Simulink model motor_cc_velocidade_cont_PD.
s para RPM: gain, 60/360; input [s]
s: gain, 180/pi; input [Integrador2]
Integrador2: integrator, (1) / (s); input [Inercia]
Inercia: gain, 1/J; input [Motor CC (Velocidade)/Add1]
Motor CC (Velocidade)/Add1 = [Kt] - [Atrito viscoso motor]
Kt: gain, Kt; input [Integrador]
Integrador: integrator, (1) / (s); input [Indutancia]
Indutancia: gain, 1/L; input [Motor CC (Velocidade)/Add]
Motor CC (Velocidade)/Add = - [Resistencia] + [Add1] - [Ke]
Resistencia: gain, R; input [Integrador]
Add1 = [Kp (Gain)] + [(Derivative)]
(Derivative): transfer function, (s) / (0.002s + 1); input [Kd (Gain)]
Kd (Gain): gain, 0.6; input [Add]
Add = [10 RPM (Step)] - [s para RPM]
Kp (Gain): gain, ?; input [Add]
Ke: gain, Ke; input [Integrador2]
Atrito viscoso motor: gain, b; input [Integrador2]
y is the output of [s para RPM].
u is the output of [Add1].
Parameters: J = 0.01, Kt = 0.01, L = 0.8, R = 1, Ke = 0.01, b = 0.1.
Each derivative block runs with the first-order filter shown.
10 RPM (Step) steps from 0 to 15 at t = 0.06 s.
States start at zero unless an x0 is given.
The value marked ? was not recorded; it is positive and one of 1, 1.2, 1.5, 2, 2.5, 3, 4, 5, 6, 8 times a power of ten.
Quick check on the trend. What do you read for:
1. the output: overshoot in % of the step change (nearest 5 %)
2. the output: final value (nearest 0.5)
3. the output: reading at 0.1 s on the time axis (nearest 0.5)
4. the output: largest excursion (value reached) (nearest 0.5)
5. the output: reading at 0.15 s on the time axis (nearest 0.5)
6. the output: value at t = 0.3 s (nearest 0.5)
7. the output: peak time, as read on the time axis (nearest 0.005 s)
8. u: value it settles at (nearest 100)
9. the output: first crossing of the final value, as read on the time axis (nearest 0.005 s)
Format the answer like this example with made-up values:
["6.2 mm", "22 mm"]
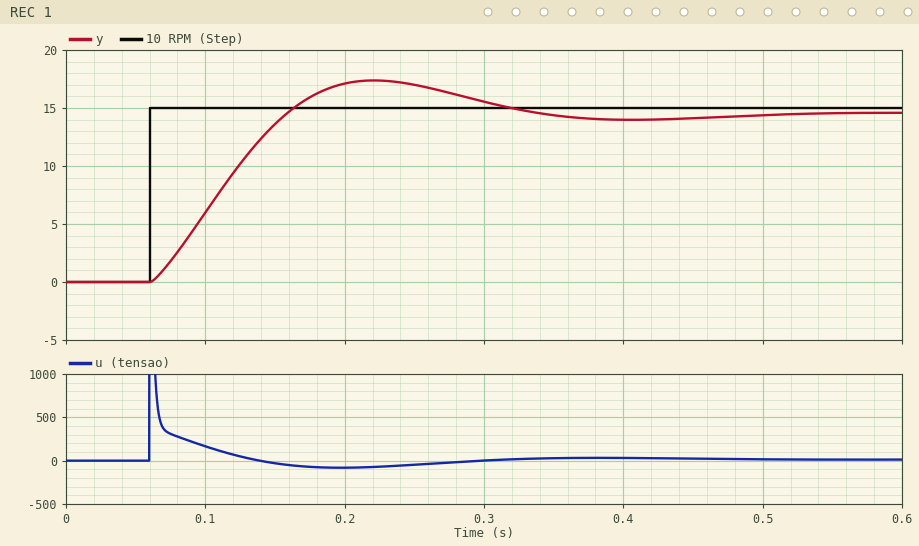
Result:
["20 %", "14.5", "6.0", "17.5", "13.5", "15.5", "0.220 s", "0", "0.160 s"]
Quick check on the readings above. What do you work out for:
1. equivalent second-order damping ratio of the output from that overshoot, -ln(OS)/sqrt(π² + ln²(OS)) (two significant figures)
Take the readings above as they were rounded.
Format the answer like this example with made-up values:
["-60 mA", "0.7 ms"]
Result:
["0.46"]
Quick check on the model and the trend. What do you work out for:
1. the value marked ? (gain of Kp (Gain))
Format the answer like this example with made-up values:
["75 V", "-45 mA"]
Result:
["30"]
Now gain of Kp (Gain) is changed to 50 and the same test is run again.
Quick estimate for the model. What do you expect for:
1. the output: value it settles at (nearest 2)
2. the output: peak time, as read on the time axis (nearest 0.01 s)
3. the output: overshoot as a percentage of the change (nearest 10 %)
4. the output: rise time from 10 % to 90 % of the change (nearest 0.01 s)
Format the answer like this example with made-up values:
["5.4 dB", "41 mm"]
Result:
["14", "0.18 s", "30 %", "0.05 s"]
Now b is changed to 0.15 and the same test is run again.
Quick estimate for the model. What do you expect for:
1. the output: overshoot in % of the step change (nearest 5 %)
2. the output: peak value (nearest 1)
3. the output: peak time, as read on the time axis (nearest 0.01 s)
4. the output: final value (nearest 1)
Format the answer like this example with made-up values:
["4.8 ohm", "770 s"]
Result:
["10 %", "16", "0.24 s", "14"]
